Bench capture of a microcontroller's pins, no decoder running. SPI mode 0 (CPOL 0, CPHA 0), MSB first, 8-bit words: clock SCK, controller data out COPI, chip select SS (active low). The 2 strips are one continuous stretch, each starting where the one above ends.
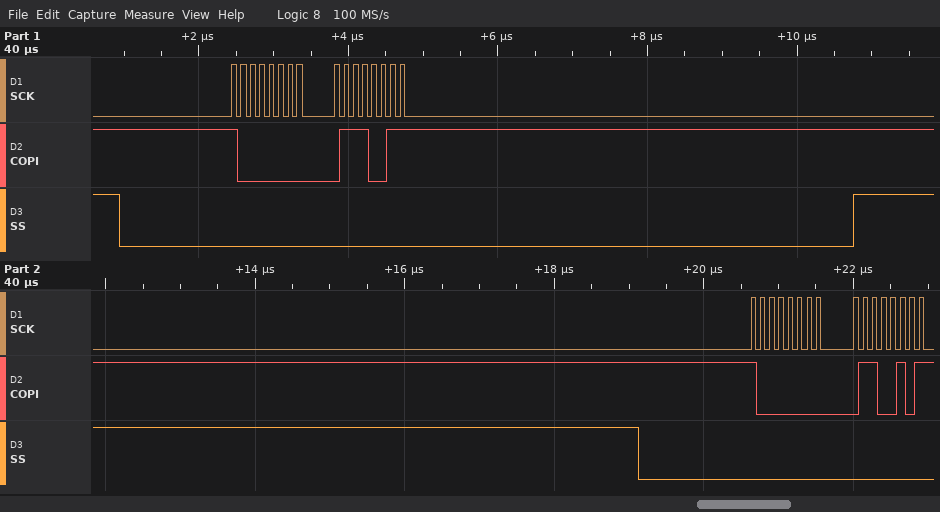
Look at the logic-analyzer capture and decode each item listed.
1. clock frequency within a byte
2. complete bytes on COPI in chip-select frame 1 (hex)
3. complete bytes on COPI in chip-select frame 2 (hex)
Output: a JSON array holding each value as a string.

["8 MHz", "80 73", "80 65"]
